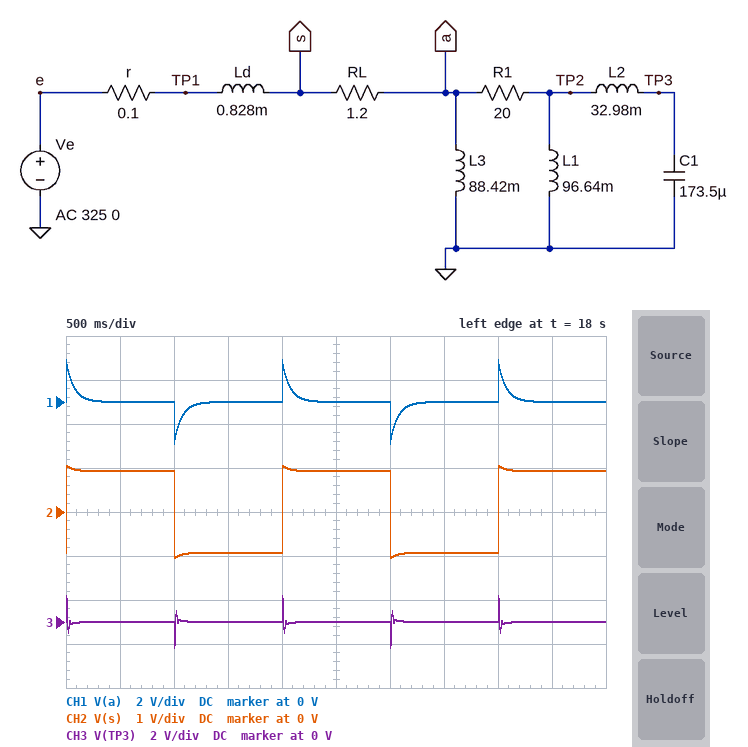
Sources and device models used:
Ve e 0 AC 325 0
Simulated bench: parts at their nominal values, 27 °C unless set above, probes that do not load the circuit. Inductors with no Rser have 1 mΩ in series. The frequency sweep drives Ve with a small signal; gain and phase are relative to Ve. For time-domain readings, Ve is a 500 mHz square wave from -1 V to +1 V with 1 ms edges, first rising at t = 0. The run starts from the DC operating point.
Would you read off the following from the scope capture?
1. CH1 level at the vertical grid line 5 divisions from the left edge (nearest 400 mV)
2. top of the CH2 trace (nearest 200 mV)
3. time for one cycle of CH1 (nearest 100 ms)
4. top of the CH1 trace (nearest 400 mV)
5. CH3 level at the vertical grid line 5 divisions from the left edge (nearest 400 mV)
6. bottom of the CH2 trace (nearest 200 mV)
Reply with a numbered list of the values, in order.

1. 0 V
2. 1.0 V
3. 2.0 s
4. 2.0 V
5. 0 V
6. -1.0 V
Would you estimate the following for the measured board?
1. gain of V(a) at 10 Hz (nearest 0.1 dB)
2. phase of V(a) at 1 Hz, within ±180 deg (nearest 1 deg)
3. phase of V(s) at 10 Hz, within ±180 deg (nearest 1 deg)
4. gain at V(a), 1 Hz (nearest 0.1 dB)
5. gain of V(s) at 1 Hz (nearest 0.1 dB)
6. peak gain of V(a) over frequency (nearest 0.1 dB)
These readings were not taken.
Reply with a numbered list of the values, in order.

1. -0.8 dB
2. 65 deg
3. 1 deg
4. -8.2 dB
5. -0.6 dB
6. -0.1 dB
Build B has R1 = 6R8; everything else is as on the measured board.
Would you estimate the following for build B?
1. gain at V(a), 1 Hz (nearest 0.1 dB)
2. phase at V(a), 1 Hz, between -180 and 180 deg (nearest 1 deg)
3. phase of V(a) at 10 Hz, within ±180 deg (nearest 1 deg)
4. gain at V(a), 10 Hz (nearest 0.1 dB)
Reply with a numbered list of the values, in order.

1. -8.5 dB
2. 63 deg
3. 16 deg
4. -1.3 dB
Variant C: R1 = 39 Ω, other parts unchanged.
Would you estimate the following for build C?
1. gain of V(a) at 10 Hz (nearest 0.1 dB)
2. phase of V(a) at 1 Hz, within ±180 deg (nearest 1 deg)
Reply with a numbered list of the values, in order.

1. -0.6 dB
2. 66 deg
